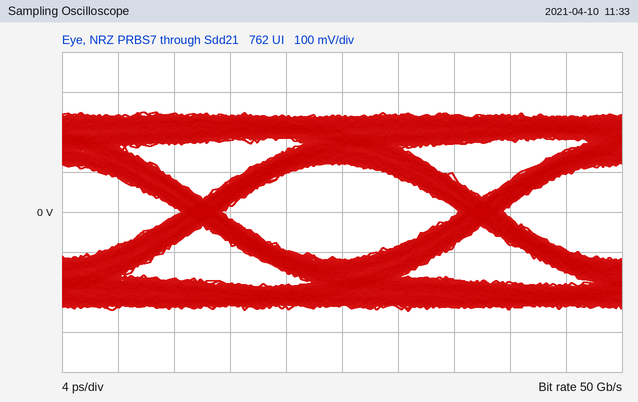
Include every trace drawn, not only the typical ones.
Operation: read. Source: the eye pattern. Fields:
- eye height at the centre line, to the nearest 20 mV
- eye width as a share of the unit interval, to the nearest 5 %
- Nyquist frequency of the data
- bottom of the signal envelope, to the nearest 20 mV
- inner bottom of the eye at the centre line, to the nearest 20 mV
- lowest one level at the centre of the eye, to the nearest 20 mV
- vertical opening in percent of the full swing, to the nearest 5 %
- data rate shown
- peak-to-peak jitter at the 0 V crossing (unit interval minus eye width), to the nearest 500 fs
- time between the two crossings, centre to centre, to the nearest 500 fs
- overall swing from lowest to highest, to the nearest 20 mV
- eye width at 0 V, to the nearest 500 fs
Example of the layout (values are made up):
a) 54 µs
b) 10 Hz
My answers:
a) 240 mV
b) 85 %
c) 25 GHz
d) -240 mV
e) -120 mV
f) 120 mV
g) 50 %
h) 50 Gb/s
i) 3.0 ps
j) 20.0 ps
k) 500 mV
l) 17.0 ps
